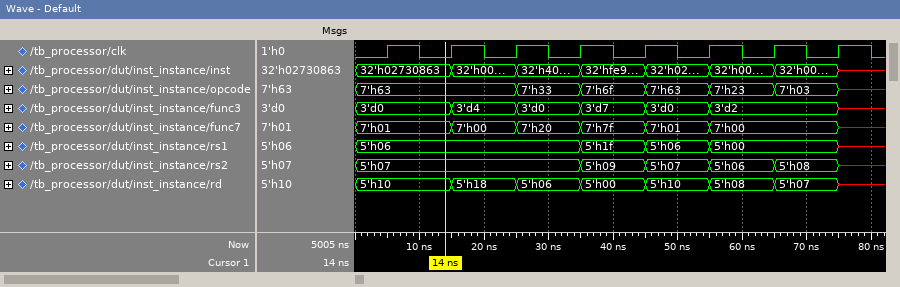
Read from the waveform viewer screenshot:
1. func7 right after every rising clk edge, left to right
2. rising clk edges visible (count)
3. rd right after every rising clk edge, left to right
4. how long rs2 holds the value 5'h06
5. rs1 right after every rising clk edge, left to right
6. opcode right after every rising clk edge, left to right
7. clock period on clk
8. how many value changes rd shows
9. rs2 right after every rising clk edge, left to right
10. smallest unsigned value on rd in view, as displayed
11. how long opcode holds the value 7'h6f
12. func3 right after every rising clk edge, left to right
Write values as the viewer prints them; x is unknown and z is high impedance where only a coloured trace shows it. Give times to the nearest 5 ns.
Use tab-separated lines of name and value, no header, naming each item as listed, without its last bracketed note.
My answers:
func7 right after every rising clk edge, left to right	7'h01, 7'h00, 7'h20, 7'h7f, 7'h01, 7'h00, 7'h00, x
rising clk edges visible	8
rd right after every rising clk edge, left to right	5'h10, 5'h18, 5'h06, 5'h00, 5'h10, 5'h08, 5'h07, x
how long rs2 holds the value 5'h06	10 ns
rs1 right after every rising clk edge, left to right	5'h06, 5'h06, 5'h06, 5'h1f, 5'h06, 5'h00, 5'h00, x
opcode right after every rising clk edge, left to right	7'h63, 7'h63, 7'h33, 7'h6f, 7'h63, 7'h23, 7'h03, x
clock period on clk	10 ns
how many value changes rd shows	7
rs2 right after every rising clk edge, left to right	5'h07, 5'h07, 5'h07, 5'h09, 5'h07, 5'h06, 5'h08, x
smallest unsigned value on rd in view, as displayed	5'h00
how long opcode holds the value 7'h6f	10 ns
func3 right after every rising clk edge, left to right	3'd0, 3'd4, 3'd0, 3'd7, 3'd0, 3'd2, 3'd2, x
